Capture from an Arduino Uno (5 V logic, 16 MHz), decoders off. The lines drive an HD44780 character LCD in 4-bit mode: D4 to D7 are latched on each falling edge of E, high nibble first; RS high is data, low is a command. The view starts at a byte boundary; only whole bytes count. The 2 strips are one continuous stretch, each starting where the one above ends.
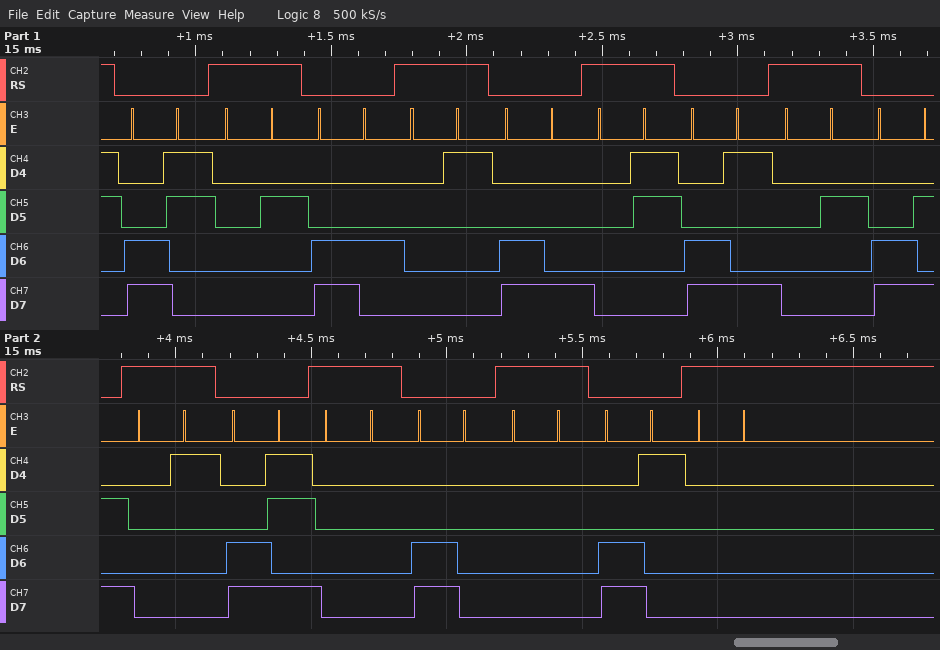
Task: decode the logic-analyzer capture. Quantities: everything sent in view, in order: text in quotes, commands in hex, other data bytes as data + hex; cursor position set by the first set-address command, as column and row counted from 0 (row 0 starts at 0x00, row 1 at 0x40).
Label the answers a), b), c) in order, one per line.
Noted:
a) 0xC3 data 02 0xC4 data 01 0xC8 data 03 0xC9 data 02 0xCA data 01 0xCB data 00 0xC0 data 00 0xC1 data 00
b) column 3, row 1
